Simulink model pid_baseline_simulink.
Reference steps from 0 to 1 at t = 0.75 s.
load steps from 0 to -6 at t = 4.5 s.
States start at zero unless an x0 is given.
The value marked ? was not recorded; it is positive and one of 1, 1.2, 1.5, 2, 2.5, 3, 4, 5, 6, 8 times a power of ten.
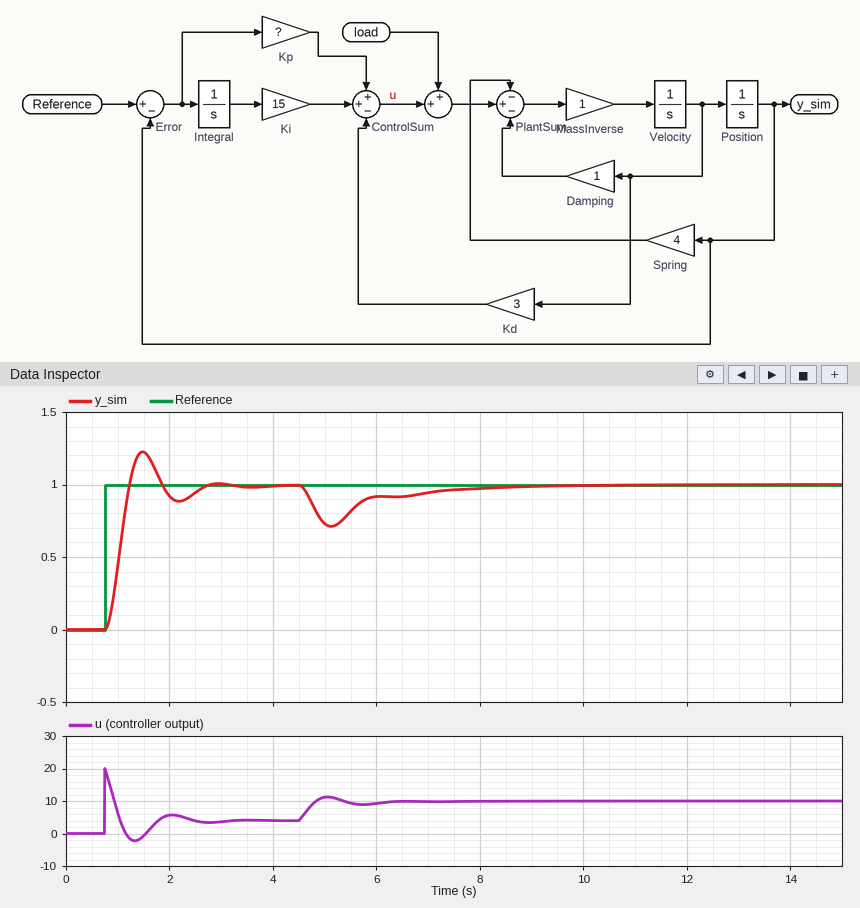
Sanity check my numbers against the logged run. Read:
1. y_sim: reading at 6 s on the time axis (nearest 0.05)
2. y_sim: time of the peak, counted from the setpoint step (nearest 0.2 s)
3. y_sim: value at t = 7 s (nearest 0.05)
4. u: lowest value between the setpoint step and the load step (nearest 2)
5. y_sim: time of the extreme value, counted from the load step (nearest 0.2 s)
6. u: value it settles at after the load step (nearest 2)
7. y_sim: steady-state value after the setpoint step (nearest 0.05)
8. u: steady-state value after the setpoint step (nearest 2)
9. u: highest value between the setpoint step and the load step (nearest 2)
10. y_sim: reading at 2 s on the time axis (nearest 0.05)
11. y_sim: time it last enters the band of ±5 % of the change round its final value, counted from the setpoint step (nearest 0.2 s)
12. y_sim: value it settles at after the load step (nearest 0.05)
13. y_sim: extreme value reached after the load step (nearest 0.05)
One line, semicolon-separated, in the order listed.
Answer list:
0.90; 0.8 s; 0.95; -2; 0.6 s; 10; 1.00; 4; 20; 0.90; 1.8 s; 1.00; 0.70
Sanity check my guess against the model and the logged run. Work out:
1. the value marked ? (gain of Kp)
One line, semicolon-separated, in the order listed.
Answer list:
20
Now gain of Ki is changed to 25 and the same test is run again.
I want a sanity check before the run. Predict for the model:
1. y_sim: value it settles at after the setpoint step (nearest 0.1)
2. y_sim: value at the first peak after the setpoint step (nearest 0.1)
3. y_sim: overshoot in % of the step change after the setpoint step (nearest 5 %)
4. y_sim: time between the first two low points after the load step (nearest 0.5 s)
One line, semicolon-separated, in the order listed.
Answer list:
1.0; 1.3; 35 %; 1.5 s
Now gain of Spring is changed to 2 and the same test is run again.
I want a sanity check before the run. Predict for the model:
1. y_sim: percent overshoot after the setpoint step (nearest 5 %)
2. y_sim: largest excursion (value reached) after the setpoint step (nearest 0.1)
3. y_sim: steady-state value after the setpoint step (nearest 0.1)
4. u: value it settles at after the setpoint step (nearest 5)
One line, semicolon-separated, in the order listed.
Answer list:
30 %; 1.3; 1.0; 0
